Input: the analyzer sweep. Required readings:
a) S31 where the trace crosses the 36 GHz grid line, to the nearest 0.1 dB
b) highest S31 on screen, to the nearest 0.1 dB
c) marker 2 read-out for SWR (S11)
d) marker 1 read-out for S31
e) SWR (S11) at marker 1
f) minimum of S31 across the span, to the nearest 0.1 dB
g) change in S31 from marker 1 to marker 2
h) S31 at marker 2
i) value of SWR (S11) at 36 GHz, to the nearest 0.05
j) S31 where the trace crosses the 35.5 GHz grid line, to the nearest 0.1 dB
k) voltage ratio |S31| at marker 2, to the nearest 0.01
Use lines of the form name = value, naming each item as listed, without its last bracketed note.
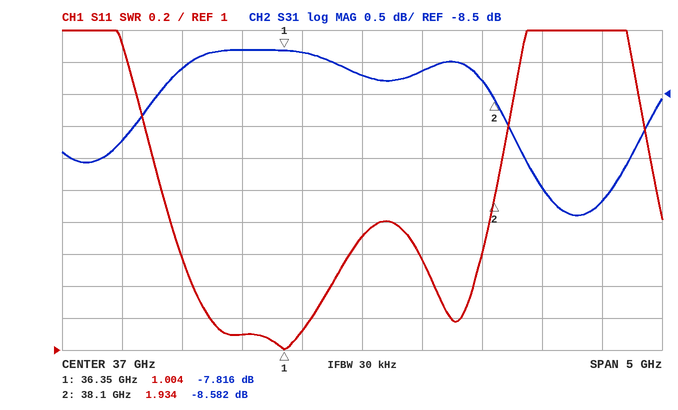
S31 where the trace crosses the 36 GHz grid line, to the nearest 0.1 dB = -7.8 dB
highest S31 on screen, to the nearest 0.1 dB = -7.8 dB
marker 2 read-out for SWR = 1.934
marker 1 read-out for S31 = -7.816 dB
SWR (S11) at marker 1 = 1.004
minimum of S31 across the span, to the nearest 0.1 dB = -10.4 dB
change in S31 from marker 1 to marker 2 = -0.766 dB
S31 at marker 2 = -8.582 dB
value of SWR (S11) at 36 GHz, to the nearest 0.05 = 1.10
S31 where the trace crosses the 35.5 GHz grid line, to the nearest 0.1 dB = -8.1 dB
voltage ratio |S31| at marker 2, to the nearest 0.01 = 0.37
